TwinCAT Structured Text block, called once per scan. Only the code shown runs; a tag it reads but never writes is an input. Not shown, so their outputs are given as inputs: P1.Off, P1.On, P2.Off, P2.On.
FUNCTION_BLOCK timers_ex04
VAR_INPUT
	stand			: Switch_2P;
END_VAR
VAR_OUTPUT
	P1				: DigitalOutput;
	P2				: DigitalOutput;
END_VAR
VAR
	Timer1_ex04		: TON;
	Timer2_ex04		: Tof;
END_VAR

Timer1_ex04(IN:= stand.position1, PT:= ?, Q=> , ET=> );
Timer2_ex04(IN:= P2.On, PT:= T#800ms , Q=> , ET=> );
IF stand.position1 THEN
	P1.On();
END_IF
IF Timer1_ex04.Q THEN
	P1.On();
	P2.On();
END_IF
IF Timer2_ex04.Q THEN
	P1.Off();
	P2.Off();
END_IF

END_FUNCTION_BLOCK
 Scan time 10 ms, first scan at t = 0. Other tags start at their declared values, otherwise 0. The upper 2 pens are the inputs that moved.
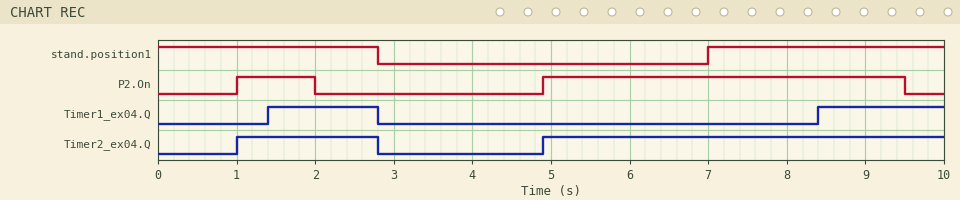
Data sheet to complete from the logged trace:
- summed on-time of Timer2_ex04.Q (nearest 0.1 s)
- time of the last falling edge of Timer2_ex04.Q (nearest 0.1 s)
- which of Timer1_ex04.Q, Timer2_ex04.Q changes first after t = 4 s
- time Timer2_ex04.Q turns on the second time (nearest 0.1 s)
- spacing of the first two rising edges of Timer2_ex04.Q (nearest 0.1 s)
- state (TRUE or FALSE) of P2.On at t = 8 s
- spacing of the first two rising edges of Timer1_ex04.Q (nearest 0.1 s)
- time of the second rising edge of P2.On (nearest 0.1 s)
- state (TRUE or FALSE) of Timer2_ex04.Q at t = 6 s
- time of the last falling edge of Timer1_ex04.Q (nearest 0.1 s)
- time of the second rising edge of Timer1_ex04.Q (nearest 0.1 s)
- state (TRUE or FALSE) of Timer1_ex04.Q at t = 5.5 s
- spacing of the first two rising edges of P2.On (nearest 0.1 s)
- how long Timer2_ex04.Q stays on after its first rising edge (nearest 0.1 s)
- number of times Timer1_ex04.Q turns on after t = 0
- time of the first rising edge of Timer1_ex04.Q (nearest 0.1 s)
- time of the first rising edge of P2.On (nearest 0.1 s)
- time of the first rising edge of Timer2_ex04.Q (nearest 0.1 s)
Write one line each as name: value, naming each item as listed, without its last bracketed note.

summed on-time of Timer2_ex04.Q: 6.9 s
time of the last falling edge of Timer2_ex04.Q: 2.8 s
which of Timer1_ex04.Q, Timer2_ex04.Q changes first after t = 4 s: Timer2_ex04.Q
time Timer2_ex04.Q turns on the second time: 4.9 s
spacing of the first two rising edges of Timer2_ex04.Q: 3.9 s
state (TRUE or FALSE) of P2.On at t = 8 s: TRUE
spacing of the first two rising edges of Timer1_ex04.Q: 7.0 s
time of the second rising edge of P2.On: 4.9 s
state (TRUE or FALSE) of Timer2_ex04.Q at t = 6 s: TRUE
time of the last falling edge of Timer1_ex04.Q: 2.8 s
time of the second rising edge of Timer1_ex04.Q: 8.4 s
state (TRUE or FALSE) of Timer1_ex04.Q at t = 5.5 s: FALSE
spacing of the first two rising edges of P2.On: 3.9 s
how long Timer2_ex04.Q stays on after its first rising edge: 1.8 s
number of times Timer1_ex04.Q turns on after t = 0: 2
time of the first rising edge of Timer1_ex04.Q: 1.4 s
time of the first rising edge of P2.On: 1.0 s
time of the first rising edge of Timer2_ex04.Q: 1.0 s
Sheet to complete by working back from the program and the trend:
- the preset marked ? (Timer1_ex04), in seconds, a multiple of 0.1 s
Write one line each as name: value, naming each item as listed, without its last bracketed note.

the preset marked ? (Timer1_ex04), in seconds, a multiple of 0.1 s: 1.4 s
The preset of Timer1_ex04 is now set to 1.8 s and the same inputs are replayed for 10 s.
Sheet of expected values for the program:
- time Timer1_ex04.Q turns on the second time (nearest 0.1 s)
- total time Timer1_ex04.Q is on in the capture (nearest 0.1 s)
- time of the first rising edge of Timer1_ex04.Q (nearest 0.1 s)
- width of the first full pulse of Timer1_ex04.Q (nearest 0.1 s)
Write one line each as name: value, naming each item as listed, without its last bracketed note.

time Timer1_ex04.Q turns on the second time: 8.8 s
total time Timer1_ex04.Q is on in the capture: 2.2 s
time of the first rising edge of Timer1_ex04.Q: 1.8 s
width of the first full pulse of Timer1_ex04.Q: 1.0 s
